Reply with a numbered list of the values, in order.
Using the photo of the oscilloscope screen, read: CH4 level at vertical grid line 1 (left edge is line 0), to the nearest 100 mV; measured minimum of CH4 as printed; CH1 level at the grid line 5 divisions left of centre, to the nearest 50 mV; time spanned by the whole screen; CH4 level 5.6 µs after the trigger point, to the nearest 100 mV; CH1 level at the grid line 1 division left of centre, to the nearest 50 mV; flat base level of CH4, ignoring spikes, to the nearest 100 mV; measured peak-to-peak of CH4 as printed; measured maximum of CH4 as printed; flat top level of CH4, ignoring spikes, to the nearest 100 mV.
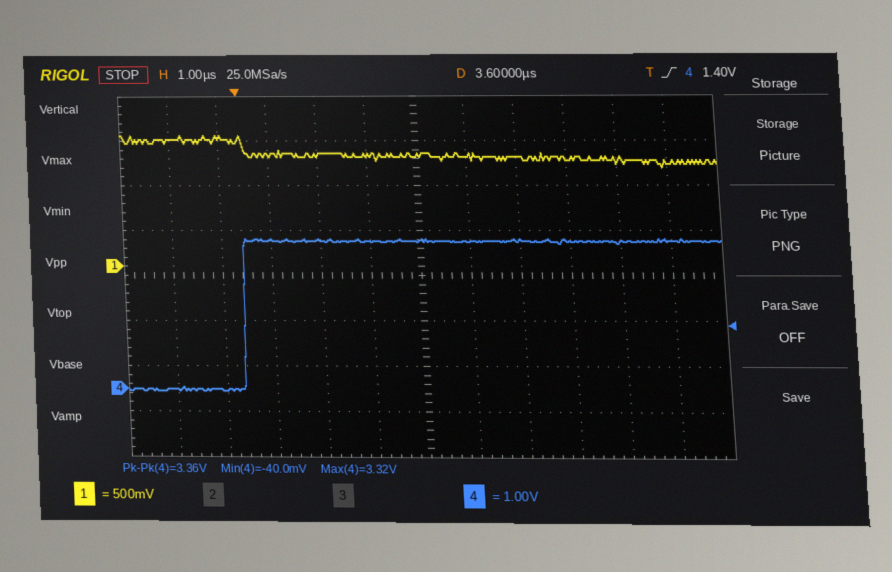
1. 0.0 V
2. -40.0 mV
3. 1.40 V
4. 12 µs
5. 3.3 V
6. 1.25 V
7. 0.0 V
8. 3.36 V
9. 3.32 V
10. 3.3 V
